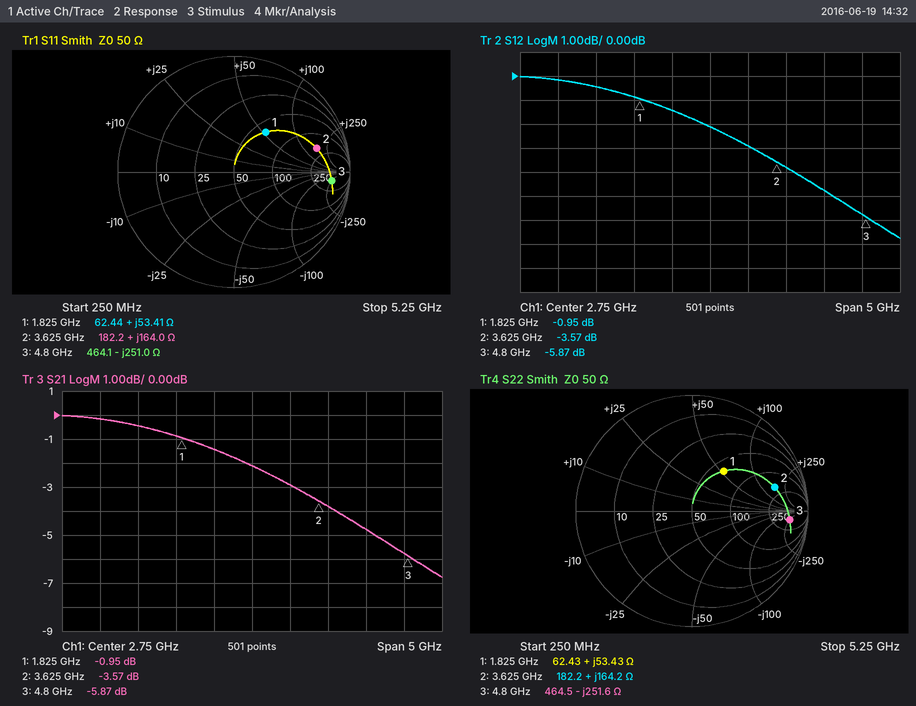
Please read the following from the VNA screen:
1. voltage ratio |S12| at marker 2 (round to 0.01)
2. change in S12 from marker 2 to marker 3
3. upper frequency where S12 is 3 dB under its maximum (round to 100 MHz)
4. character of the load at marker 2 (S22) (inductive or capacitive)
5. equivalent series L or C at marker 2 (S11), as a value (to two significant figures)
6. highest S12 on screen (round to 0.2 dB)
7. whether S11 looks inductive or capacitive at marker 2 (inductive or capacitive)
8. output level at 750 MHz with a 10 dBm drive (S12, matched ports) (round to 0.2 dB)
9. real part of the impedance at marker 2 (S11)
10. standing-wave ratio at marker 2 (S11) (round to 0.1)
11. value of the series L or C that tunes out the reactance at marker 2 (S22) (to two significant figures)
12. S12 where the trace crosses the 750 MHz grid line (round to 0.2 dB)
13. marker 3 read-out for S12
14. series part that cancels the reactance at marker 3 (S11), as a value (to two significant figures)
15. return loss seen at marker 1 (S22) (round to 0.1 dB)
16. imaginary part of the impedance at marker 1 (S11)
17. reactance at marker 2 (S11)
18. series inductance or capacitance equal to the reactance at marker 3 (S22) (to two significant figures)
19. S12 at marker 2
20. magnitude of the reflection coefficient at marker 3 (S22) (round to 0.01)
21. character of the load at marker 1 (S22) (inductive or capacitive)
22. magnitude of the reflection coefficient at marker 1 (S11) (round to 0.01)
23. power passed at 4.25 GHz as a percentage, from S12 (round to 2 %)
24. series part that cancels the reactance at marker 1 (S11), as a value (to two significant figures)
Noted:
0.66
-2.30 dB
3.3 GHz
inductive
7.2 nH
0.0 dB
inductive
9.8 dBm
182.2 Ω
6.7
270 fF
-0.2 dB
-5.87 dB
8.3 nH
7.1 dB
+53.41 Ω
+164.0 Ω
130 fF
-3.57 dB
0.85
inductive
0.44
34 %
1.6 pF
